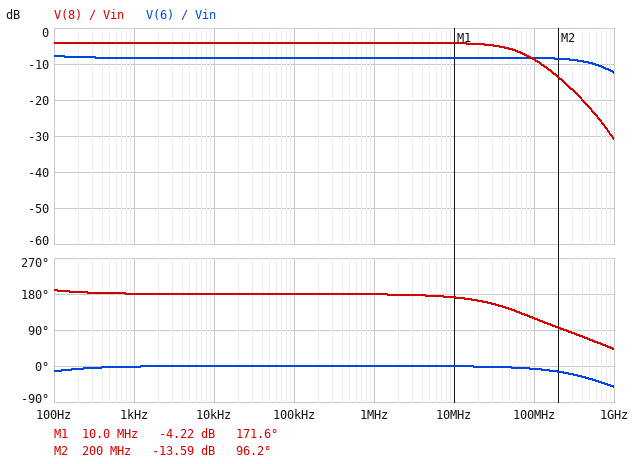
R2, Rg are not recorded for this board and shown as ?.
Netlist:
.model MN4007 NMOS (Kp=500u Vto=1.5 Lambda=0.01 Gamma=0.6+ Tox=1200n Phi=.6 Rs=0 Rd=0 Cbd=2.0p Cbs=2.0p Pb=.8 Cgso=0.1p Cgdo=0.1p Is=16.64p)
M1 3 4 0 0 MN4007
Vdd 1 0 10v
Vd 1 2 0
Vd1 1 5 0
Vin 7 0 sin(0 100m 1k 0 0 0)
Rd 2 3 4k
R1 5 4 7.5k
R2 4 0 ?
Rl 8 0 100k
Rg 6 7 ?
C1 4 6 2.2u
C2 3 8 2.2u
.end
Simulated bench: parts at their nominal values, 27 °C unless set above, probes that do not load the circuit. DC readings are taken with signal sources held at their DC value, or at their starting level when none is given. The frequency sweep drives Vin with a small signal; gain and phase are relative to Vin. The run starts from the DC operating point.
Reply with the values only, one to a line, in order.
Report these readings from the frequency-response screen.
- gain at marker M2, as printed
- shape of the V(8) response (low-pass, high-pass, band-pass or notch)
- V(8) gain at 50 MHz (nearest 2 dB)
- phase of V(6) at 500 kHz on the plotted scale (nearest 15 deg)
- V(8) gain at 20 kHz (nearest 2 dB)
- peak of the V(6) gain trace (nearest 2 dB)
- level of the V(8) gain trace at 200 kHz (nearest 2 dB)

-13.59 dB
low-pass
-6 dB
0 deg
-4 dB
-8 dB
-4 dB
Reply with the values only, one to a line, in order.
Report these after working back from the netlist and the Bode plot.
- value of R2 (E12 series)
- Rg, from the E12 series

2.2 kΩ
2.7 kΩ
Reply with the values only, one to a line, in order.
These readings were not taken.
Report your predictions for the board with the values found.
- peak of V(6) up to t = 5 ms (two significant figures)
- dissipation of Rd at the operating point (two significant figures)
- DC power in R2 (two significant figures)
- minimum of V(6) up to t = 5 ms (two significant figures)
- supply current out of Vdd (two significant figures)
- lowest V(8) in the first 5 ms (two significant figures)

40 mV
100 µW
2.3 mW
-38 mV
1.2 mA
-63 mV
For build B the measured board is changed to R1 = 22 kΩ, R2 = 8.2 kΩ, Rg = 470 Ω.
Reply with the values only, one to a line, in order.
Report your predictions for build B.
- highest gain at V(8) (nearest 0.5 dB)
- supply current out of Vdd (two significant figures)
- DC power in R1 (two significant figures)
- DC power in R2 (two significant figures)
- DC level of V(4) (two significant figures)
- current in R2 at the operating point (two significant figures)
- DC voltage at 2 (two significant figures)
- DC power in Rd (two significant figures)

7.5 dB
730 µA
2.4 mW
900 µW
2.7 V
330 µA
10 V
640 µW
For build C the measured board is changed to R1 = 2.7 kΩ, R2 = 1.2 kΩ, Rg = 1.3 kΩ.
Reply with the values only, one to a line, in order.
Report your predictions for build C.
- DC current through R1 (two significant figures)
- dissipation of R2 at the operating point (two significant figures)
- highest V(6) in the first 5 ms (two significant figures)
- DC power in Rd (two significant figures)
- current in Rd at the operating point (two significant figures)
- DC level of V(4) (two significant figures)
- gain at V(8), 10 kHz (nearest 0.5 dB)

2.6 mA
7.9 mW
41 mV
1.8 mW
670 µA
3.1 V
2.0 dB
